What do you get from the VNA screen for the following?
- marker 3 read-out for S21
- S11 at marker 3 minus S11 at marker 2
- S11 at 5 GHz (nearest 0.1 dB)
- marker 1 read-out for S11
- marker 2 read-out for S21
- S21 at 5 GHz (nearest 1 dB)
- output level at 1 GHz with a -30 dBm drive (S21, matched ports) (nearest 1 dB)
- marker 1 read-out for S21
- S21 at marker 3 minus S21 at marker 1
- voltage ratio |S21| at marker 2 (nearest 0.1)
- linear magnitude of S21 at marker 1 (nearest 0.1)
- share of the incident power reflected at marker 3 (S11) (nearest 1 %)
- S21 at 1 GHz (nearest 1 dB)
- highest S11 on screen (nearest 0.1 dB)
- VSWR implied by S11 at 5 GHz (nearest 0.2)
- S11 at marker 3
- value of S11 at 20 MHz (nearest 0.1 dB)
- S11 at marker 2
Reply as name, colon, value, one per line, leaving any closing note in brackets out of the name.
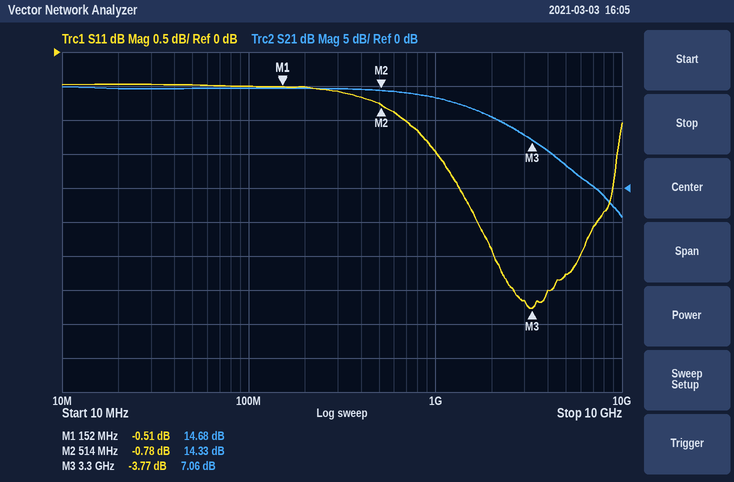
marker 3 read-out for S21: 7.06 dB
S11 at marker 3 minus S11 at marker 2: -2.99 dB
S11 at 5 GHz: -3.3 dB
marker 1 read-out for S11: -0.51 dB
marker 2 read-out for S21: 14.33 dB
S21 at 5 GHz: 3 dB
output level at 1 GHz with a -30 dBm drive (S21, matched ports): -17 dBm
marker 1 read-out for S21: 14.68 dB
S21 at marker 3 minus S21 at marker 1: -7.62 dB
voltage ratio |S21| at marker 2: 5.2
linear magnitude of S21 at marker 1: 5.4
share of the incident power reflected at marker 3 (S11): 42 %
S21 at 1 GHz: 13 dB
highest S11 on screen: -0.5 dB
VSWR implied by S11 at 5 GHz: 5.4
S11 at marker 3: -3.77 dB
value of S11 at 20 MHz: -0.5 dB
S11 at marker 2: -0.78 dB
